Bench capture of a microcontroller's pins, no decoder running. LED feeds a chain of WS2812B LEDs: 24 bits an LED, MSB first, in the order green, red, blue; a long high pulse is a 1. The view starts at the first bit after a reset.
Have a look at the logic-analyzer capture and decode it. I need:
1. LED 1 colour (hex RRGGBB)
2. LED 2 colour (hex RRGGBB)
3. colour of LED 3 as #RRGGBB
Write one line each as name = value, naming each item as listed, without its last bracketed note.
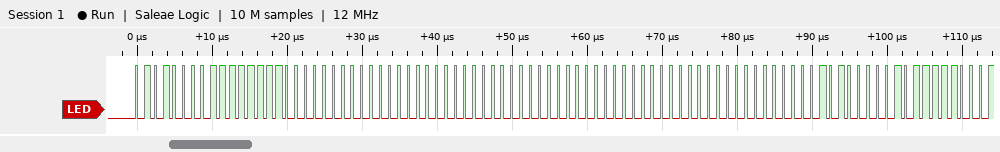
LED 1 colour = #FF5000
LED 2 colour = #000000
colour of LED 3 as #RRGGBB = #000000
